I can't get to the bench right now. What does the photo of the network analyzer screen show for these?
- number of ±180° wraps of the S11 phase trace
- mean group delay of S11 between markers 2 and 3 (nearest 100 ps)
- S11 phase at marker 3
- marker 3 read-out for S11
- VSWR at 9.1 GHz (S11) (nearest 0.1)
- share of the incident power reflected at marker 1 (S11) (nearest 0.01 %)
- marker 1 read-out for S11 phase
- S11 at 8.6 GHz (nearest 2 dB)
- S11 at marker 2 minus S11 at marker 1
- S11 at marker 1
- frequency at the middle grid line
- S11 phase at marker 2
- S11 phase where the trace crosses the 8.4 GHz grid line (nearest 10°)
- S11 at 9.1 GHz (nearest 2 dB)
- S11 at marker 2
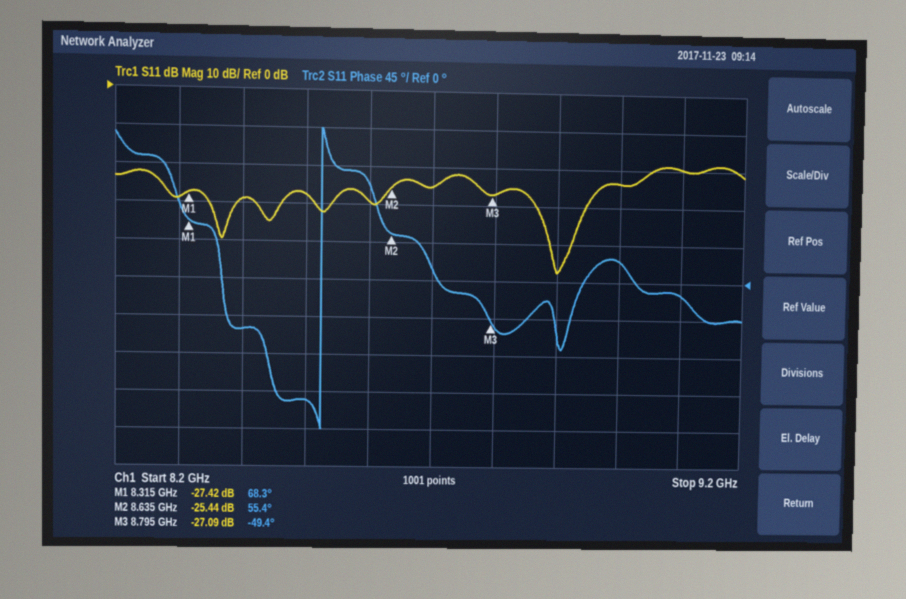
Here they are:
1
1.8 ns
-49.4°
-27.09 dB
1.2
0.18 %
68.3°
-30 dB
1.98 dB
-27.42 dB
8.7 GHz
55.4°
-60°
-20 dB
-25.44 dB
